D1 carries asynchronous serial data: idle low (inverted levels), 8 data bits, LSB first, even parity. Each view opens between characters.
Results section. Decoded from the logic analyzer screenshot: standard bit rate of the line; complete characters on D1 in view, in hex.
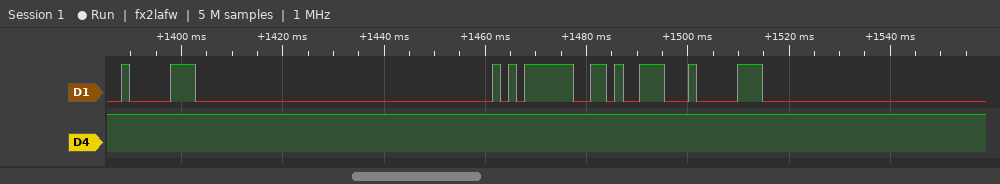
600 baud
1F, 05, 1A, 1F
